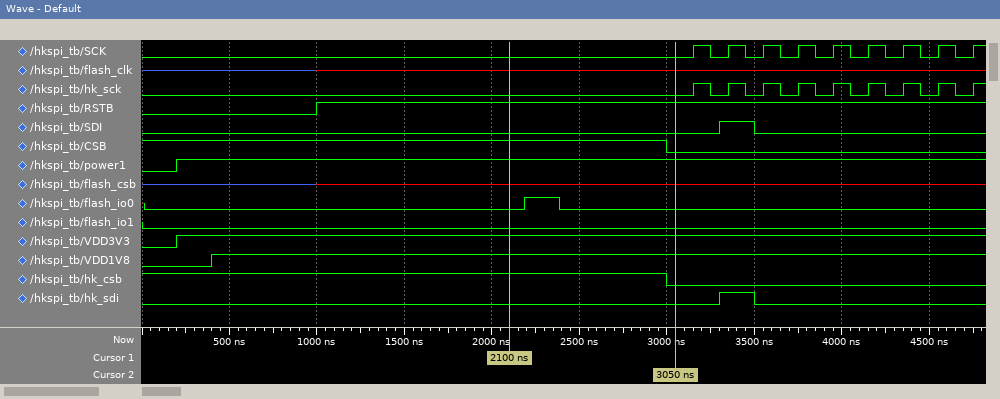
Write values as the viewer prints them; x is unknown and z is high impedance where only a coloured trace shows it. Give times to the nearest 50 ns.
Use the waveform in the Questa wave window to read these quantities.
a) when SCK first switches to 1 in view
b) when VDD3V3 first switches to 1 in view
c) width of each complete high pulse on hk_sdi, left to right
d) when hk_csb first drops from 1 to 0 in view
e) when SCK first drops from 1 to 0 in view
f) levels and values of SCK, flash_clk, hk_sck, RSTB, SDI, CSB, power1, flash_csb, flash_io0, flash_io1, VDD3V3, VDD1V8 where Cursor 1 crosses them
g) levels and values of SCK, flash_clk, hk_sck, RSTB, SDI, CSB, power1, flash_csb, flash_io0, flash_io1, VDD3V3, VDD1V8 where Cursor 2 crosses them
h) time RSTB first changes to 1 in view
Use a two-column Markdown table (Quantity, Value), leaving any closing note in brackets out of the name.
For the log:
| Quantity | Value |
|---|---|
| when SCK first switches to 1 in view | 3150 ns |
| when VDD3V3 first switches to 1 in view | 200 ns |
| width of each complete high pulse on hk_sdi, left to right | 200 ns |
| when hk_csb first drops from 1 to 0 in view | 3000 ns |
| when SCK first drops from 1 to 0 in view | 3250 ns |
| levels and values of SCK, flash_clk, hk_sck, RSTB, SDI, CSB, power1, flash_csb, flash_io0, flash_io1, VDD3V3, VDD1V8 where Cursor 1 crosses them | SCK=0, flash_clk=x, hk_sck=0, RSTB=1, SDI=0, CSB=1, power1=1, flash_csb=x, flash_io0=0, flash_io1=0, VDD3V3=1, VDD1V8=1 |
| levels and values of SCK, flash_clk, hk_sck, RSTB, SDI, CSB, power1, flash_csb, flash_io0, flash_io1, VDD3V3, VDD1V8 where Cursor 2 crosses them | SCK=0, flash_clk=x, hk_sck=0, RSTB=1, SDI=0, CSB=0, power1=1, flash_csb=x, flash_io0=0, flash_io1=0, VDD3V3=1, VDD1V8=1 |
| time RSTB first changes to 1 in view | 1000 ns |
